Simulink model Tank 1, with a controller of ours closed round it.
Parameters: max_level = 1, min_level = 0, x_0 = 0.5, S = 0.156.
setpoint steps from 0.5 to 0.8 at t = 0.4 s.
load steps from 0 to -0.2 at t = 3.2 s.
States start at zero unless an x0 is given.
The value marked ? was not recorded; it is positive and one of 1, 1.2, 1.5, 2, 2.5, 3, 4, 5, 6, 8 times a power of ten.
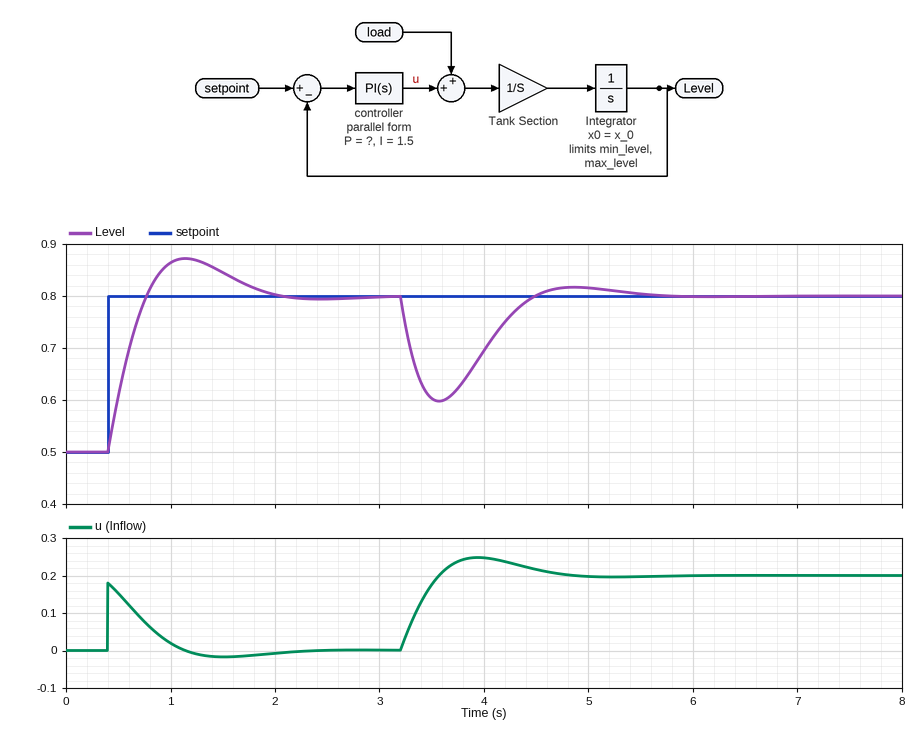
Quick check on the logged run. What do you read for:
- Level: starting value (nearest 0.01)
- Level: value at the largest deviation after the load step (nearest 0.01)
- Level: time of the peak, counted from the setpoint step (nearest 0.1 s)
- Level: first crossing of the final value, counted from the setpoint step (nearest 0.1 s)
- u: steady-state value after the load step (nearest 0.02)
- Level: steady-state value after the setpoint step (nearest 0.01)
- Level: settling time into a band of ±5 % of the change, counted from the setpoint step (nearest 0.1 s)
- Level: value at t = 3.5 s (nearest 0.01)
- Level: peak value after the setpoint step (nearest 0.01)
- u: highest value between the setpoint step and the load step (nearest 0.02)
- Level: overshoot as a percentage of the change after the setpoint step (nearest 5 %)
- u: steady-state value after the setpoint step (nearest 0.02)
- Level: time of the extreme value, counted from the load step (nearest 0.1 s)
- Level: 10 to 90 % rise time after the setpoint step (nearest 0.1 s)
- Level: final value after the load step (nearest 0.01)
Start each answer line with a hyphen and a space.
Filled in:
- 0.50
- 0.60
- 0.7 s
- 0.4 s
- 0.20
- 0.80
- 1.4 s
- 0.60
- 0.87
- 0.18
- 25 %
- 0.00
- 0.4 s
- 0.3 s
- 0.80
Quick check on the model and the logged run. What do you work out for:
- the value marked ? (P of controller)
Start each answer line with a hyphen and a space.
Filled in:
- 0.6
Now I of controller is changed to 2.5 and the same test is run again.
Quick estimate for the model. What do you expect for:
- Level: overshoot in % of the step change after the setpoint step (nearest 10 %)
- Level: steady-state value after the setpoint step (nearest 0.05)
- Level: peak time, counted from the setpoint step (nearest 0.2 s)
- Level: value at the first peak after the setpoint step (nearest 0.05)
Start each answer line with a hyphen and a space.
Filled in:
- 30 %
- 0.80
- 0.6 s
- 0.90
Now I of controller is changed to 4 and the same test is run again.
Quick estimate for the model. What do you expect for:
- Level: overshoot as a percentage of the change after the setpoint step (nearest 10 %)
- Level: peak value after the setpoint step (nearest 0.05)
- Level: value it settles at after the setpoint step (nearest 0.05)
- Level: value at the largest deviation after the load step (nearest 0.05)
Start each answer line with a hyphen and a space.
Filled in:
- 40 %
- 0.90
- 0.80
- 0.65
